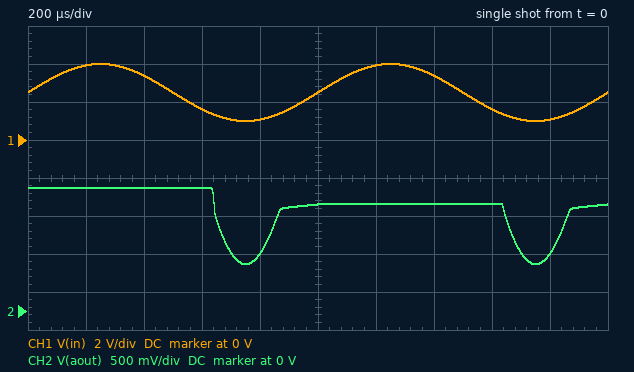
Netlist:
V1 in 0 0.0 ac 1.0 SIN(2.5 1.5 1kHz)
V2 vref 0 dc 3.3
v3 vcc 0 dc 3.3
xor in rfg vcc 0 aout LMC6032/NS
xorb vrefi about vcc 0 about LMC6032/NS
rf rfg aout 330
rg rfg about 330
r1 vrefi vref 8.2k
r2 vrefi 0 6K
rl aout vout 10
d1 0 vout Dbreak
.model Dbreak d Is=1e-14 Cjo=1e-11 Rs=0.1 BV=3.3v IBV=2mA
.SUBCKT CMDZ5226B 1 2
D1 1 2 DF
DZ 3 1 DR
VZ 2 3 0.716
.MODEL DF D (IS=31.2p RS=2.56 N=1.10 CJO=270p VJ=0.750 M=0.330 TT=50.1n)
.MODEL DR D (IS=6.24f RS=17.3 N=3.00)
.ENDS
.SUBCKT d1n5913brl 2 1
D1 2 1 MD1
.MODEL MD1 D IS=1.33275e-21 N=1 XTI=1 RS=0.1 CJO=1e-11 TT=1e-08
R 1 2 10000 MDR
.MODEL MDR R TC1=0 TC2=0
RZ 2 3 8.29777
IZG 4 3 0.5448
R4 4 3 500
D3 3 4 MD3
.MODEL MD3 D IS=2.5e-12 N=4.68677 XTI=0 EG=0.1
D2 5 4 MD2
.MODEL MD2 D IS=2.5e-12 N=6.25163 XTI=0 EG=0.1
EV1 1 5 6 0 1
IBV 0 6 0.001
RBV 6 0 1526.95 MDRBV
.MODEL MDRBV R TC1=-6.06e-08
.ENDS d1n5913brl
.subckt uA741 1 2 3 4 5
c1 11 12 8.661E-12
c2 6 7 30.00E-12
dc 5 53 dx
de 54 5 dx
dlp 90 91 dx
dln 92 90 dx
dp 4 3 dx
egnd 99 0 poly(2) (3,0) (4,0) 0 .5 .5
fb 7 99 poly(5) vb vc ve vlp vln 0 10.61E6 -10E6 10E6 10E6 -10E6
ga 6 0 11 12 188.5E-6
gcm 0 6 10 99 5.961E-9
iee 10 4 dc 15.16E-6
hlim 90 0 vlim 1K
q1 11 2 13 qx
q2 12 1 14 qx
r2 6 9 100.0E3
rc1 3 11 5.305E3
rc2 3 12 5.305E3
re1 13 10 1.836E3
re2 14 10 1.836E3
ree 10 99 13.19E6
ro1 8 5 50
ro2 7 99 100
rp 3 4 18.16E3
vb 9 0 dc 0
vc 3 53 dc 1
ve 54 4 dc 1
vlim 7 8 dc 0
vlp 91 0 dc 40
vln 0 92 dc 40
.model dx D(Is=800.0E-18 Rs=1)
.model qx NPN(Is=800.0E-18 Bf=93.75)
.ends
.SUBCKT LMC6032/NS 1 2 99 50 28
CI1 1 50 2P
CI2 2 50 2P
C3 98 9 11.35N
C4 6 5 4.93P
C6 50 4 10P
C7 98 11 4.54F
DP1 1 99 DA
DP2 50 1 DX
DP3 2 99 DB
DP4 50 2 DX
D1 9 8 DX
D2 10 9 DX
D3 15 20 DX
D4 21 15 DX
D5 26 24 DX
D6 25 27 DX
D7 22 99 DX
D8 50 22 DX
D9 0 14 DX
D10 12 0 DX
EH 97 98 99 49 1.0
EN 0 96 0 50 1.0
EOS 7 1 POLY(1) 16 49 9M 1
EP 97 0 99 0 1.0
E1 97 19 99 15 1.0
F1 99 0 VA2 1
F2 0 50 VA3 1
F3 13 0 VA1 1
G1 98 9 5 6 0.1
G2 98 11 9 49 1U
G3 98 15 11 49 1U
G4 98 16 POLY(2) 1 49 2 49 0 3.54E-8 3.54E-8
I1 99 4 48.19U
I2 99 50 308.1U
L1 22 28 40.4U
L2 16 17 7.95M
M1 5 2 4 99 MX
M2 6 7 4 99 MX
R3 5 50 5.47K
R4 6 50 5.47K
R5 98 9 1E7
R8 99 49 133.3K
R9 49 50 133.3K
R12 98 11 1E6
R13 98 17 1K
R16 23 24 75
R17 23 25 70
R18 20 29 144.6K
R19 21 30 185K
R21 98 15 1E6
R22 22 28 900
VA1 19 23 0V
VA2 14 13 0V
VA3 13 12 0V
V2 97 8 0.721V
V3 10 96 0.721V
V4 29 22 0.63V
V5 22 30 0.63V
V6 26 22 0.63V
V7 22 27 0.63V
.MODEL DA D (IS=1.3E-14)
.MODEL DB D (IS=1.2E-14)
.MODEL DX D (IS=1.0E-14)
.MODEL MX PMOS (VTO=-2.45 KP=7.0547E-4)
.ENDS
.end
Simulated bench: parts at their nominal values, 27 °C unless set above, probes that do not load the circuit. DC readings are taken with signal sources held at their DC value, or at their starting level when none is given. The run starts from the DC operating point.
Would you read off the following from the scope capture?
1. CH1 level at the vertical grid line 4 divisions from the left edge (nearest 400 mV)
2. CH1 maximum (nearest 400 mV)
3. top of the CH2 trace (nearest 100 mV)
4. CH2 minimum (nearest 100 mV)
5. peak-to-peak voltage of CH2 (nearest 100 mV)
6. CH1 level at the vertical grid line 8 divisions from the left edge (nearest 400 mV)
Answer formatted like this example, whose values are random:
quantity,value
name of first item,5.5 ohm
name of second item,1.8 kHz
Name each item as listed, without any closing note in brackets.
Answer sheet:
quantity,value
CH1 level at the vertical grid line 4 divisions from the left edge,1.2 V
CH1 maximum,4.0 V
top of the CH2 trace,1.6 V
CH2 minimum,600 mV
peak-to-peak voltage of CH2,1.0 V
CH1 level at the vertical grid line 8 divisions from the left edge,1.6 V
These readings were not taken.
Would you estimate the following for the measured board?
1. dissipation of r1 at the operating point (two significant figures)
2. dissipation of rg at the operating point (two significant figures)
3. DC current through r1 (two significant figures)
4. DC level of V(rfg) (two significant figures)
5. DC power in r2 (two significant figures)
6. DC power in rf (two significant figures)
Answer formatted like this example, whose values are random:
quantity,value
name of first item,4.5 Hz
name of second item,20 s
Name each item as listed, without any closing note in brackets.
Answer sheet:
quantity,value
dissipation of r1 at the operating point,440 µW
dissipation of rg at the operating point,1.2 mW
DC current through r1,230 µA
DC level of V(rfg),780 mV
DC power in r2,320 µW
DC power in rf,1.2 mW
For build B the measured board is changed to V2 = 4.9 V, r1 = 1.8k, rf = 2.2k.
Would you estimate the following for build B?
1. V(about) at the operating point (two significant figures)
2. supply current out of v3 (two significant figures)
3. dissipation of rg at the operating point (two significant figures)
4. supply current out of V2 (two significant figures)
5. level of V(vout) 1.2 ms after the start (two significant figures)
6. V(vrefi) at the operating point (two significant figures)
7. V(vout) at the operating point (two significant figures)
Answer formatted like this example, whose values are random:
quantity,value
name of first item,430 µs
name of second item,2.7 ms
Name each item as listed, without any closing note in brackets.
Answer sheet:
quantity,value
V(about) at the operating point,1.6 V
supply current out of v3,1.3 mA
dissipation of rg at the operating point,120 µW
supply current out of V2,630 µA
level of V(vout) 1.2 ms after the start,300 mV
V(vrefi) at the operating point,3.8 V
V(vout) at the operating point,43 mV
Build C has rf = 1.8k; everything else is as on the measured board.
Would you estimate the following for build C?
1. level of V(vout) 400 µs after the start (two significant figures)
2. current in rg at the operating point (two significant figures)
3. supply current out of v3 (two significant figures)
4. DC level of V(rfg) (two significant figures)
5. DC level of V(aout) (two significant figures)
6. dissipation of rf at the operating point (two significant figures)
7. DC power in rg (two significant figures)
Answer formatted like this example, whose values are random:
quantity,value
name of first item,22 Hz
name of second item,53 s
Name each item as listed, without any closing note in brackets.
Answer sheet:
quantity,value
level of V(vout) 400 µs after the start,1.6 V
current in rg at the operating point,640 µA
supply current out of v3,1.3 mA
DC level of V(rfg),1.2 V
DC level of V(aout),46 mV
dissipation of rf at the operating point,730 µW
DC power in rg,130 µW
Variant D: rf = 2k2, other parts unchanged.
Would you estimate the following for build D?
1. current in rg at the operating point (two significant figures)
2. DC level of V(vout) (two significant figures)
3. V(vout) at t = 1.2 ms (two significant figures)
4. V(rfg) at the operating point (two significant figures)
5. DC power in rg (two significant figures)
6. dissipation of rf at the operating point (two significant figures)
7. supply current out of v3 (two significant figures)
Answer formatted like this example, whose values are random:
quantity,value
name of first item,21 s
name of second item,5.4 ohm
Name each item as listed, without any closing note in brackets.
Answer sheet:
quantity,value
current in rg at the operating point,540 µA
DC level of V(vout),36 mV
V(vout) at t = 1.2 ms,1.4 V
V(rfg) at the operating point,1.2 V
DC power in rg,96 µW
dissipation of rf at the operating point,640 µW
supply current out of v3,1.2 mA
